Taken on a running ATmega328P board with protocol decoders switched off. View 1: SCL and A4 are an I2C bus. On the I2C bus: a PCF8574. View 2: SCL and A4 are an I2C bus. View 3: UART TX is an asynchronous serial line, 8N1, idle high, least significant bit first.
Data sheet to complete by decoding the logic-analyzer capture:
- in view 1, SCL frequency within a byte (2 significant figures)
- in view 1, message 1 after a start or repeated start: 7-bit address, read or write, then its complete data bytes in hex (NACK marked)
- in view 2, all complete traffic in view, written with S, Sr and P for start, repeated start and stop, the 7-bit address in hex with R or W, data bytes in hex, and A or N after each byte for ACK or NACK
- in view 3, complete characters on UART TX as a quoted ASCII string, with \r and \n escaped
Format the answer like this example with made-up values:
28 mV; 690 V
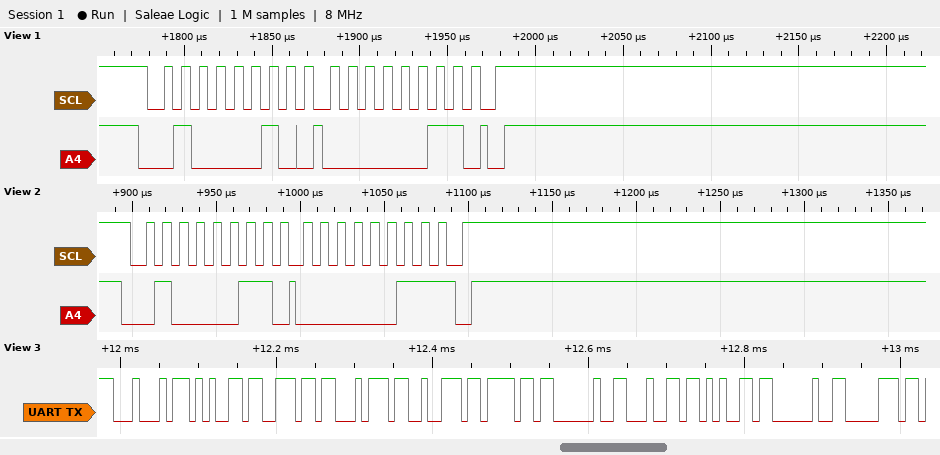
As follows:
100 kHz; 0x21 write: 03; S 21R A 03 N P; "Dentro de p"
